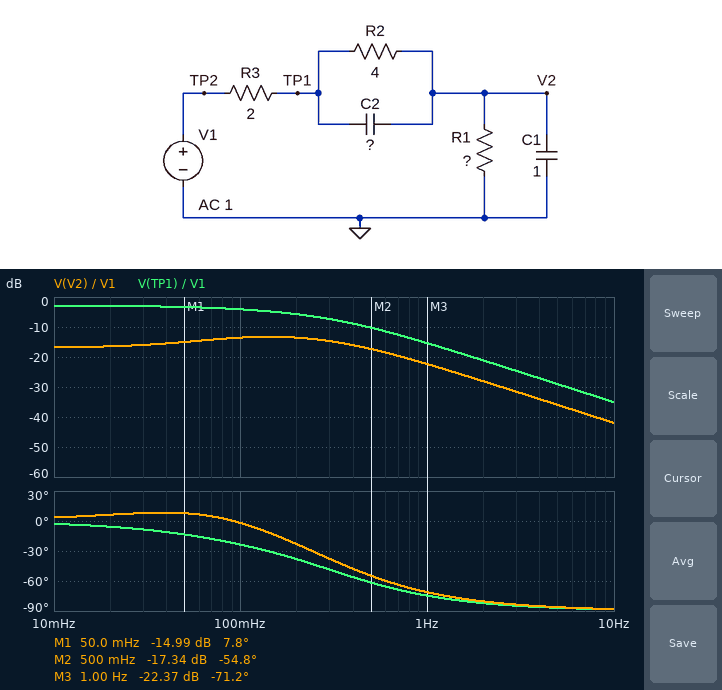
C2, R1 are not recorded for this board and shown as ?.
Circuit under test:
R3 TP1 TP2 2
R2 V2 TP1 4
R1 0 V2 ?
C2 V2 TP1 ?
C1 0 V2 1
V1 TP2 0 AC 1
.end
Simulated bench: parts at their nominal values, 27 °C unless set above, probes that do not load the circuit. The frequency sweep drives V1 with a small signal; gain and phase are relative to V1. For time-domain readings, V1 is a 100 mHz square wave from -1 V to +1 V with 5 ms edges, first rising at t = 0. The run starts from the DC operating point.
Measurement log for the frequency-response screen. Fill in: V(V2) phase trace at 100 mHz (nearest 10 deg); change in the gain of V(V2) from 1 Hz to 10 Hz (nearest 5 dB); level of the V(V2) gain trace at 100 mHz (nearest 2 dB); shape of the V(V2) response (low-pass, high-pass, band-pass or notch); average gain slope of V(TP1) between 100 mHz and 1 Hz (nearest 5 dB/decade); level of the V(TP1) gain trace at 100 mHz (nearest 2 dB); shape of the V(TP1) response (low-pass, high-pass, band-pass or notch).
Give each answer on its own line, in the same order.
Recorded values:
0 deg
-20 dB
-14 dB
low-pass
-10 dB/decade
-4 dB
low-pass
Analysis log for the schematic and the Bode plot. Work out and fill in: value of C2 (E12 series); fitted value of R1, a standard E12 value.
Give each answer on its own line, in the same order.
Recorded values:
820 mF
1 Ω
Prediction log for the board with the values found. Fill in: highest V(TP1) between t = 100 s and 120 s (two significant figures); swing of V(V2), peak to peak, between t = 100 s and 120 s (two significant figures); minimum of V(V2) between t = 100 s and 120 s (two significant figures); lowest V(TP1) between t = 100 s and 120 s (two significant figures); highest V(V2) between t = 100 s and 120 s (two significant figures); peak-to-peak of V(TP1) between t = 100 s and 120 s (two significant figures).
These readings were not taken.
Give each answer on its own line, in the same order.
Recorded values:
700 mV
500 mV
-250 mV
-700 mV
250 mV
1.4 V
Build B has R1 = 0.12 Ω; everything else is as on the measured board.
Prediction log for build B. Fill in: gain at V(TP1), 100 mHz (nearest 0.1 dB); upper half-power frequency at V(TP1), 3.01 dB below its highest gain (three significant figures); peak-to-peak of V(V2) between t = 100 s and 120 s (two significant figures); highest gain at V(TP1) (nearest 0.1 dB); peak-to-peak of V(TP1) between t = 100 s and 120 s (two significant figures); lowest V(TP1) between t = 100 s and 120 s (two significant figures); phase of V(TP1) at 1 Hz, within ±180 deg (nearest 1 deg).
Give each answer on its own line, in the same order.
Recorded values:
-5.2 dB
143 mHz
150 mV
-3.4 dB
1.3 V
-660 mV
-64 deg
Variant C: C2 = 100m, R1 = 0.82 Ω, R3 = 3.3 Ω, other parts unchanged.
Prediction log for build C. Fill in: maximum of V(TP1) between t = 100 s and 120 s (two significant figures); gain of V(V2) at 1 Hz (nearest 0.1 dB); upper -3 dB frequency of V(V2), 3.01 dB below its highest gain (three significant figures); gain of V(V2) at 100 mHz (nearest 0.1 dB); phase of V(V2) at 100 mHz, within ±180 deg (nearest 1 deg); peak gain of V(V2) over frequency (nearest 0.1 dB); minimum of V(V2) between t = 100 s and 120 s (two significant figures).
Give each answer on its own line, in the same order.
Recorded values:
590 mV
-28.5 dB
270 mHz
-20.6 dB
-18 deg
-19.9 dB
-100 mV
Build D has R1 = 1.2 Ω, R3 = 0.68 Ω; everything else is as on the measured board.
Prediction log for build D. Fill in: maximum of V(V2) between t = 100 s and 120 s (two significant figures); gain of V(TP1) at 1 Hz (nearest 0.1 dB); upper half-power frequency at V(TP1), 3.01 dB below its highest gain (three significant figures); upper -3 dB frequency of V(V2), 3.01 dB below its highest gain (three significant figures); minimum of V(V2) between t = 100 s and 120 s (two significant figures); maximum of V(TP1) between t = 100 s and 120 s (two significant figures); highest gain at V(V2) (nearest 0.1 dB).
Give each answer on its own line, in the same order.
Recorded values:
420 mV
-7.1 dB
566 mHz
746 mHz
-420 mV
880 mV
-9.3 dB
